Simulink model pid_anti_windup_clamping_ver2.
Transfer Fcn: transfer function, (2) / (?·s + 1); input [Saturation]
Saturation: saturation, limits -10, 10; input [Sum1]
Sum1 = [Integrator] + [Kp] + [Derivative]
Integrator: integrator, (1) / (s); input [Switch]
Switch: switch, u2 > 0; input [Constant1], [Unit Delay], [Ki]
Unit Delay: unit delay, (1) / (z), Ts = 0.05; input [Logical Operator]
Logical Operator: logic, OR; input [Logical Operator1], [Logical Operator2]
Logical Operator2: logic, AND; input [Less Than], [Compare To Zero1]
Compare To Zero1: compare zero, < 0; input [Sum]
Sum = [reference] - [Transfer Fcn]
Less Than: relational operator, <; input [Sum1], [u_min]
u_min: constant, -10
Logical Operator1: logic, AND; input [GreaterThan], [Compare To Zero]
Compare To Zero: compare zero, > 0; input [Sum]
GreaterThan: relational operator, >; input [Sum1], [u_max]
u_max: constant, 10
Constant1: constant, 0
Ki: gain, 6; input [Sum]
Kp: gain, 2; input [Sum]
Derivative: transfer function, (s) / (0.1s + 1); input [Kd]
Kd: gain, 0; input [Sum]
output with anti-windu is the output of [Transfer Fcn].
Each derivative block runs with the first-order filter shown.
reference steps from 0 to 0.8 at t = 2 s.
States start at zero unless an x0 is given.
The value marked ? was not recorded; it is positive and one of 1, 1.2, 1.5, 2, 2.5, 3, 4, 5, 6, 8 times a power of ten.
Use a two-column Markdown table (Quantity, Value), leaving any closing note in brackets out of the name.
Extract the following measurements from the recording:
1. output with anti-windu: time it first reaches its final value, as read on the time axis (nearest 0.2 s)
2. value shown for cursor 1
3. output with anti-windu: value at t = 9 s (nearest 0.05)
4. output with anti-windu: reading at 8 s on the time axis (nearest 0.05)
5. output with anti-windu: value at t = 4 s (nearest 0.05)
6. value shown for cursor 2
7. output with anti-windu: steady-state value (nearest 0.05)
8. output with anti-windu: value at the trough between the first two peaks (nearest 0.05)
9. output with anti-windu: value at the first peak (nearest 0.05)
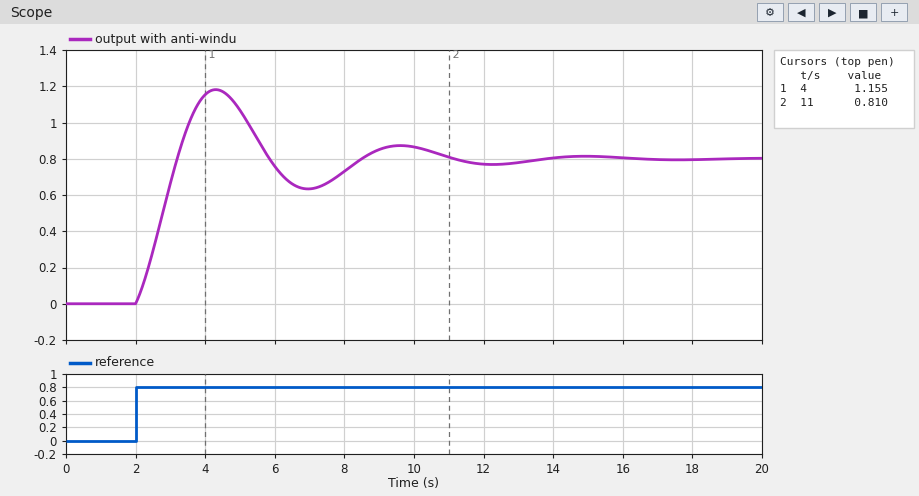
| Quantity | Value |
|---|---|
| output with anti-windu: time it first reaches its final value, as read on the time axis | 3.2 s |
| value shown for cursor 1 | 1.155 |
| output with anti-windu: value at t = 9 s | 0.85 |
| output with anti-windu: reading at 8 s on the time axis | 0.75 |
| output with anti-windu: value at t = 4 s | 1.15 |
| value shown for cursor 2 | 0.810 |
| output with anti-windu: steady-state value | 0.80 |
| output with anti-windu: value at the trough between the first two peaks | 0.65 |
| output with anti-windu: value at the first peak | 1.20 |
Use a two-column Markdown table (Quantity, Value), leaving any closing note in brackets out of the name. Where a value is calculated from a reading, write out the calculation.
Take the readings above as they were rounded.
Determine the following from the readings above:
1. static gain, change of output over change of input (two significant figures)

| Quantity | Value |
|---|---|
| static gain, change of output over change of input | (0.8 - 0) / (0.8 - 0) = 1.0 |
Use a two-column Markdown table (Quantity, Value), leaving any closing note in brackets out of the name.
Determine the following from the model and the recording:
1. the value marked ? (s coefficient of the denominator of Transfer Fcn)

| Quantity | Value |
|---|---|
| the value marked ? | 8 |
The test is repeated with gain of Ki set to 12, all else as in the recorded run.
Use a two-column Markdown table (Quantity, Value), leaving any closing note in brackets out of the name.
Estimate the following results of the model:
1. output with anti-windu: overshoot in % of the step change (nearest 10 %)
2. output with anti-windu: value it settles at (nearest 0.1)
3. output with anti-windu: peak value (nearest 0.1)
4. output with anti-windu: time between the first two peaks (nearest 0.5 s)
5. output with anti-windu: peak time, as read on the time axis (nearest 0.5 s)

| Quantity | Value |
|---|---|
| output with anti-windu: overshoot in % of the step change | 60 % |
| output with anti-windu: value it settles at | 0.8 |
| output with anti-windu: peak value | 1.3 |
| output with anti-windu: time between the first two peaks | 3.5 s |
| output with anti-windu: peak time, as read on the time axis | 3.5 s |
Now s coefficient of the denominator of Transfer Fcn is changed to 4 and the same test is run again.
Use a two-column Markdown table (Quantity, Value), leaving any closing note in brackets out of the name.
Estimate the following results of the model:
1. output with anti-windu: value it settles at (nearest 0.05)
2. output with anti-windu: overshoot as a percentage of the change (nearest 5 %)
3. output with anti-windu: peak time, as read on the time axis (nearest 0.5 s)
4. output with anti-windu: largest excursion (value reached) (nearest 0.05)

| Quantity | Value |
|---|---|
| output with anti-windu: value it settles at | 0.80 |
| output with anti-windu: overshoot as a percentage of the change | 35 % |
| output with anti-windu: peak time, as read on the time axis | 3.5 s |
| output with anti-windu: largest excursion (value reached) | 1.10 |
